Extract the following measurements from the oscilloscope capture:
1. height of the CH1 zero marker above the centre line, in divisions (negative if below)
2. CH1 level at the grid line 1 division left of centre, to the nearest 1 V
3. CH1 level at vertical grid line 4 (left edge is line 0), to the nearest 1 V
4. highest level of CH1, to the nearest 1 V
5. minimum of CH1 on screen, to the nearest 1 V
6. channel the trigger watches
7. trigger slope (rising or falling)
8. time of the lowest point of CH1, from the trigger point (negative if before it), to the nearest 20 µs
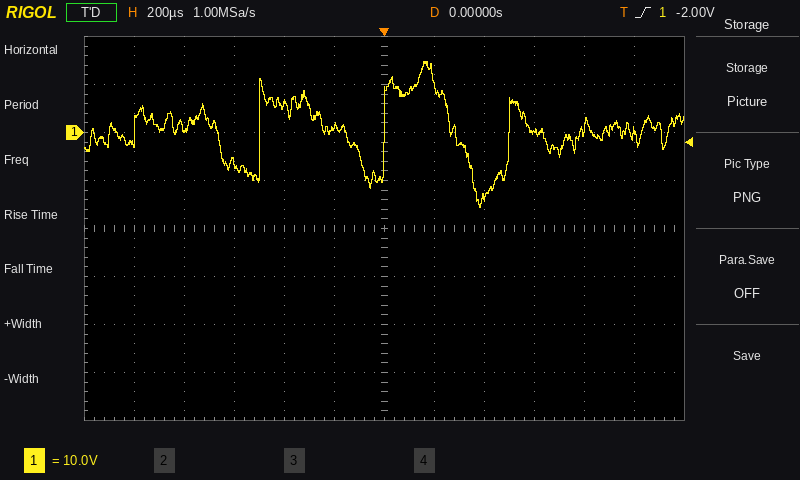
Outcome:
+2.0 div
1 V
6 V
15 V
-16 V
CH1
rising
+380 µs
